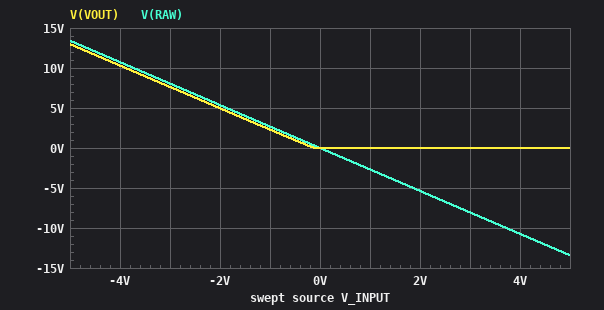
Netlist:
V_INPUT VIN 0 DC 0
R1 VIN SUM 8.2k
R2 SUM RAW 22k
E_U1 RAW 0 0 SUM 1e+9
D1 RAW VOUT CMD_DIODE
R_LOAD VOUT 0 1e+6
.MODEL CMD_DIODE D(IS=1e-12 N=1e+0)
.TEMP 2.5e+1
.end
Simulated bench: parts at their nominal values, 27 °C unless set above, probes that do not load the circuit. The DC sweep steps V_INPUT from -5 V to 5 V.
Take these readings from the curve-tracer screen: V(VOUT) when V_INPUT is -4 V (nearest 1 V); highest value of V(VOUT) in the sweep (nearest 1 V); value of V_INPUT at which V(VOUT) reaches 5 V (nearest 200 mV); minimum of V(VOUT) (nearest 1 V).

10 V
13 V
-2.0 V
0 V
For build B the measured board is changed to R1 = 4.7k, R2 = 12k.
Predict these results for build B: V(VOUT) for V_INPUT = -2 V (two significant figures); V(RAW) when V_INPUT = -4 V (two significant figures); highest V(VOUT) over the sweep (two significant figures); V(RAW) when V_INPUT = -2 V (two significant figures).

4.7 V
10 V
12 V
5.1 V
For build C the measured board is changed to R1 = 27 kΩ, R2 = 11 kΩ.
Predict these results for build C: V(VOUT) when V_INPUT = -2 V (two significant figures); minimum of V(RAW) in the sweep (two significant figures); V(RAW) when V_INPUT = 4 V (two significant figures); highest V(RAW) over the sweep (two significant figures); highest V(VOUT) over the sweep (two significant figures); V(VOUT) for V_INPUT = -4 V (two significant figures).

470 mV
-2.0 V
-1.6 V
2.0 V
1.7 V
1.3 V
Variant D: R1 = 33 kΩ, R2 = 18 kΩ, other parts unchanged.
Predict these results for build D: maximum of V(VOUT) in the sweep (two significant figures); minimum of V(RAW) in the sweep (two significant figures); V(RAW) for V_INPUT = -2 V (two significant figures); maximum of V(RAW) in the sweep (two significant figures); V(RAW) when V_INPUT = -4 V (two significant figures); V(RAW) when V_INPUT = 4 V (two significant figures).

2.3 V
-2.7 V
1.1 V
2.7 V
2.2 V
-2.2 V
